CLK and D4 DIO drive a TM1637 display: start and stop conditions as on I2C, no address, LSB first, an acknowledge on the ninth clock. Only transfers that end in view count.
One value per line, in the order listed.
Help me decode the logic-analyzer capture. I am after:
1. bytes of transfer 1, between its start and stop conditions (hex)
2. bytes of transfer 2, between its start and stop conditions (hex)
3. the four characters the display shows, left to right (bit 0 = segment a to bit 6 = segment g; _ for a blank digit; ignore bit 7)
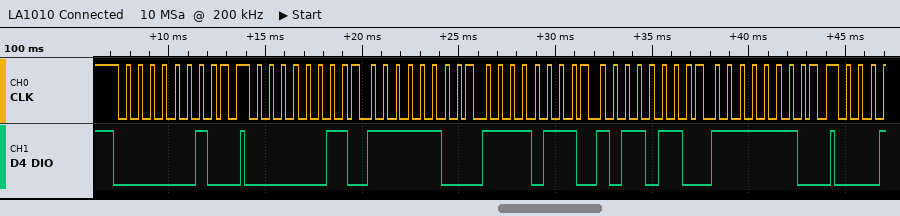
40
C0 3F EF 6D 7F
0958
